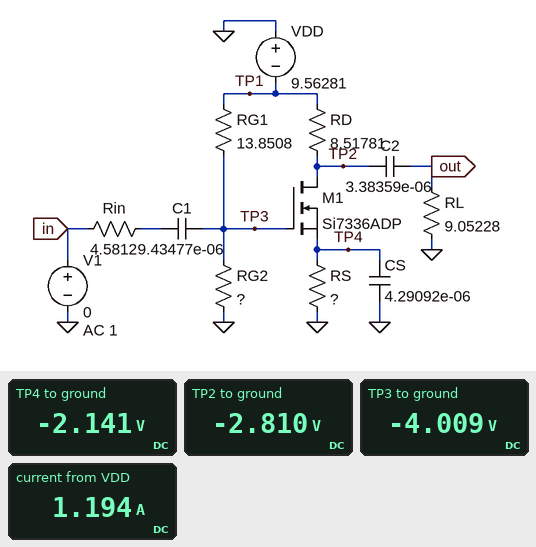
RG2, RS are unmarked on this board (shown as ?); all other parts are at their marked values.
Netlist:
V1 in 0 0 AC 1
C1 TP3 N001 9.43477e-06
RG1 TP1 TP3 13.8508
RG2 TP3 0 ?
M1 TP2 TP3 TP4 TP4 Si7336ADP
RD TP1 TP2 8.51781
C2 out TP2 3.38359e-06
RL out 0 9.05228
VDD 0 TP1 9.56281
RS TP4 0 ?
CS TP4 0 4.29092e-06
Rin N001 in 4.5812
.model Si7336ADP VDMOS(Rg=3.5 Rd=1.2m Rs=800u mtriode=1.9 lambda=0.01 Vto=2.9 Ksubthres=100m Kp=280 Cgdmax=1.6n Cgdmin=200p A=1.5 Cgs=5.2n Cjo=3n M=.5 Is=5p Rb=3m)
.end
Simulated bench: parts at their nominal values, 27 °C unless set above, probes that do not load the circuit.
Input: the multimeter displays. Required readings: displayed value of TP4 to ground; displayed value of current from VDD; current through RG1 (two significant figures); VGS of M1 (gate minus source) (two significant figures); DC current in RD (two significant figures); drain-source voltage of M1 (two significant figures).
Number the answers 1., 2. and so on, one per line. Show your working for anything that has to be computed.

1. -2.141 V
2. 1.194 A
3. (-4.009 V - (-9.563 V)) / 13.85 Ω = 400 mA
4. -4.009 V - (-2.141 V) = -1.9 V
5. (-2.81 V - (-9.563 V)) / 8.518 Ω = 790 mA
6. -2.81 V - (-2.141 V) = -670 mV
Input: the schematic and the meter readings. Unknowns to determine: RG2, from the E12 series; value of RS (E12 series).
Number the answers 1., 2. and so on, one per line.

1. 10 Ω
2. 2.7 Ω
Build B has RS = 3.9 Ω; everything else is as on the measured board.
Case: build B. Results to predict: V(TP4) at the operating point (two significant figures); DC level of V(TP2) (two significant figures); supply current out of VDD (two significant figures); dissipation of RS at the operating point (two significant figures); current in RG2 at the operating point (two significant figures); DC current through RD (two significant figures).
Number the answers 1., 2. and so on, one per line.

1. -2.8 V
2. -3.5 V
3. 1.1 A
4. 2.0 W
5. 400 mA
6. 720 mA
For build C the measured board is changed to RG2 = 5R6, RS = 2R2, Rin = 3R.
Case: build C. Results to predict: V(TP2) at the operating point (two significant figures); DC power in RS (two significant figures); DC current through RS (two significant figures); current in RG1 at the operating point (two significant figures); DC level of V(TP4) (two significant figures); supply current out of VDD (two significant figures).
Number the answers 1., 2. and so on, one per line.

1. -2.5 V
2. 1.5 W
3. 830 mA
4. 490 mA
5. -1.8 V
6. 1.3 A
